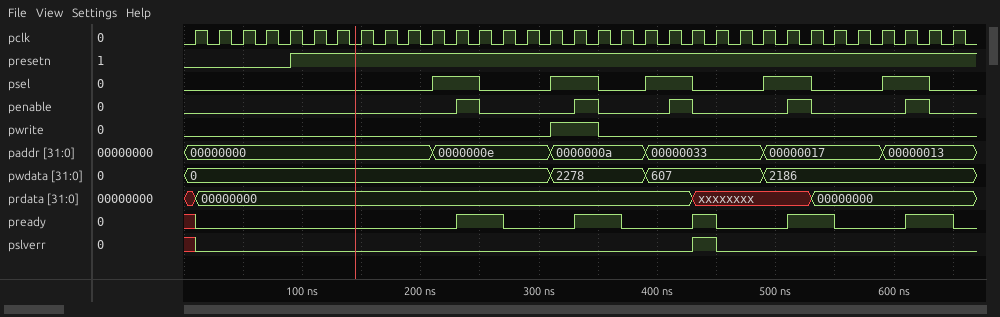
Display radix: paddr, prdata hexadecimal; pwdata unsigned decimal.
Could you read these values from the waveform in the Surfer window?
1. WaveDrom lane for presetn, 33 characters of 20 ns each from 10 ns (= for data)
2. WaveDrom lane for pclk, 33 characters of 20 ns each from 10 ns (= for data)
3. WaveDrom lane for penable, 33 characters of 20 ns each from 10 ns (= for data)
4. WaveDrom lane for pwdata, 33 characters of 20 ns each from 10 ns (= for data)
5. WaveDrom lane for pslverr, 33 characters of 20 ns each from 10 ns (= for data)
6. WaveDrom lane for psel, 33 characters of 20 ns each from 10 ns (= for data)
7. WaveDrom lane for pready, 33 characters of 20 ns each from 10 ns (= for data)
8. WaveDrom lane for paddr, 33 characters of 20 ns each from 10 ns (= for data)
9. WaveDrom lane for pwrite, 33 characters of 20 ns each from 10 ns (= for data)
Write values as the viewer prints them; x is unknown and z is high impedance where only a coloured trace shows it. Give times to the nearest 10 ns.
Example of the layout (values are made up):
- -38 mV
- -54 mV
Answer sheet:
- {name: 'presetn', wave: '0...1............................'}
- {name: 'pclk', wave: 'p................................'}
- {name: 'penable', wave: '0..........10...10..10...10...10.'}
- {name: 'pwdata', wave: '=..............=...=....=........', data: '0 2278 607 2186'}
- {name: 'pslverr', wave: '0....................10..........'}
- {name: 'psel', wave: '0.........1.0..1.0.1.0..1.0..1.0.'}
- {name: 'pready', wave: '0..........1.0..1.0..10..1.0..1.0'}
- {name: 'paddr', wave: '=.........=....=...=....=....=...', data: '00000000 0000000e 0000000a 00000033 00000017 00000013'}
- {name: 'pwrite', wave: '0..............1.0...............'}
